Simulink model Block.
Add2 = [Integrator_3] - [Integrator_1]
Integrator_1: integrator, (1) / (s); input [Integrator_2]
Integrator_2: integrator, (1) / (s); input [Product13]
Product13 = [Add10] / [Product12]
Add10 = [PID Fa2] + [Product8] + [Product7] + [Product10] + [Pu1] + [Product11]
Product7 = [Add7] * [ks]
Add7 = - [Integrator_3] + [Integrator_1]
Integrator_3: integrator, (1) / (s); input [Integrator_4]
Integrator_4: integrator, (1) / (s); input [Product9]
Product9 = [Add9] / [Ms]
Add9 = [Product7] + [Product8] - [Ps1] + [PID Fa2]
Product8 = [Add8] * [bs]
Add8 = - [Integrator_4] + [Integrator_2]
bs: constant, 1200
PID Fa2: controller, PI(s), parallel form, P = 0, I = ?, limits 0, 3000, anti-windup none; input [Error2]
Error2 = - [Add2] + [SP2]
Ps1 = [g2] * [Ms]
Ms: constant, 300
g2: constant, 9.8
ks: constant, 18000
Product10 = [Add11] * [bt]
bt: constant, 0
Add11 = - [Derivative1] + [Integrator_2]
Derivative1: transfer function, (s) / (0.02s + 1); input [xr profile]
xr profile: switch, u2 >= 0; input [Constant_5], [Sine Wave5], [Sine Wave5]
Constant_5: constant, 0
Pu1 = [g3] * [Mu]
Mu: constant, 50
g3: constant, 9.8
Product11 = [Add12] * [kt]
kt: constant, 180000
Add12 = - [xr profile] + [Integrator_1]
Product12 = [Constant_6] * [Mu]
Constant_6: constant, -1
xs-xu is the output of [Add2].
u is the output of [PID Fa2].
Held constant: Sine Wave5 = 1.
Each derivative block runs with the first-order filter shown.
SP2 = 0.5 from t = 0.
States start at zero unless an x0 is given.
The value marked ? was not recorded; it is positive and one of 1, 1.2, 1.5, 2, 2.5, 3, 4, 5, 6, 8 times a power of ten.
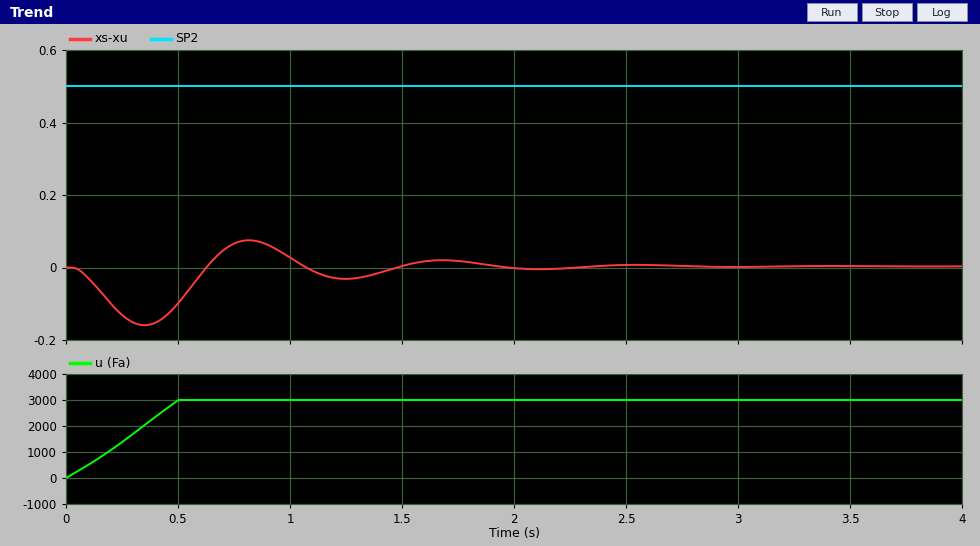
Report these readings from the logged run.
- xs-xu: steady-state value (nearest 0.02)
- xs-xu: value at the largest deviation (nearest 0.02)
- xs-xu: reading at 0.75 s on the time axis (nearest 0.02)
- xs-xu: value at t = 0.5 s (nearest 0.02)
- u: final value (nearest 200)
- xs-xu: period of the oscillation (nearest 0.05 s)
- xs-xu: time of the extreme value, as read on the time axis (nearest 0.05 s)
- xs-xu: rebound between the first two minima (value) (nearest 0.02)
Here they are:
0.00
-0.16
0.06
-0.10
3000
0.90 s
0.35 s
0.08
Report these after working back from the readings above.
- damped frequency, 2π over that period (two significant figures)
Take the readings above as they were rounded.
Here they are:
7.0 rad/s
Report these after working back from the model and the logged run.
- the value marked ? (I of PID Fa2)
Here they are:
10000
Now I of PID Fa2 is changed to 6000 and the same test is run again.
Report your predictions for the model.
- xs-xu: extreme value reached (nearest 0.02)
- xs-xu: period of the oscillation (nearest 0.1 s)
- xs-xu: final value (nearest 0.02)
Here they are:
-0.18
1.0 s
0.00
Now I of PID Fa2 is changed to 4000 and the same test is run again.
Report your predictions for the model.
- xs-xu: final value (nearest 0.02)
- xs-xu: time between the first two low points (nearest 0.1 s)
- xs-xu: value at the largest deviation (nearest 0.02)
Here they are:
0.00
0.8 s
-0.20
